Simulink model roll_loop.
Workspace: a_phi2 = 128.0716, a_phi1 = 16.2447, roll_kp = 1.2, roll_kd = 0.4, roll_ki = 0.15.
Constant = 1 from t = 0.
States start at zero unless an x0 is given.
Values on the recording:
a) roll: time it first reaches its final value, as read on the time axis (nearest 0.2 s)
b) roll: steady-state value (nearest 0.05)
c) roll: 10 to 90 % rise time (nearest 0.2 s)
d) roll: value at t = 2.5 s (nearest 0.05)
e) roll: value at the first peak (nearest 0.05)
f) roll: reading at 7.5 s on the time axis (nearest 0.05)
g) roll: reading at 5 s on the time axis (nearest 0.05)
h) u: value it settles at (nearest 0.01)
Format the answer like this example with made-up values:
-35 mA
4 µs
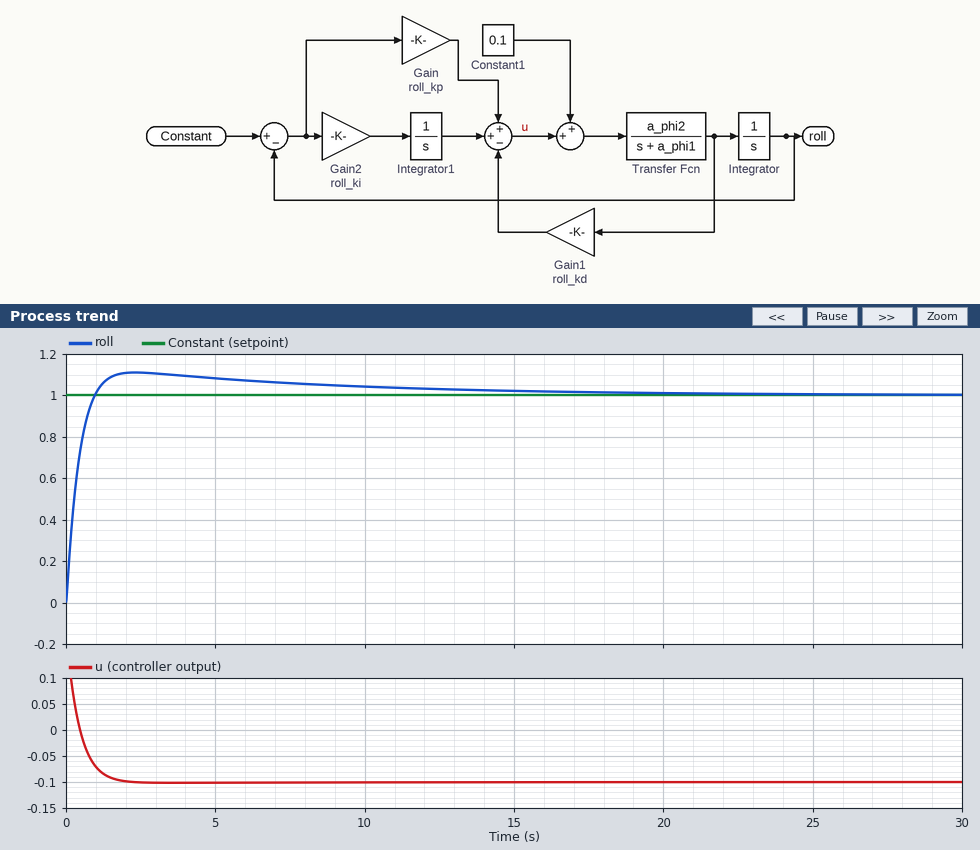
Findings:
1.0 s
1.00
0.6 s
1.10
1.10
1.05
1.10
-0.10
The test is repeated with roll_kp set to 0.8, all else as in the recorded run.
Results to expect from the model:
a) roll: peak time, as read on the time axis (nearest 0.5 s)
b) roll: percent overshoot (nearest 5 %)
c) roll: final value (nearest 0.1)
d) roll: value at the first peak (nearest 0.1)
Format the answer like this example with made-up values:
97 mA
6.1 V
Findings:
3.0 s
15 %
1.0
1.2
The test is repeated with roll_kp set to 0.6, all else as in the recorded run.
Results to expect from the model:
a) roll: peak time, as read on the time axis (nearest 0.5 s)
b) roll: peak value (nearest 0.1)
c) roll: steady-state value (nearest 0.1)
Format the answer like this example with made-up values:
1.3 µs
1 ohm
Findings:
3.0 s
1.2
1.0
